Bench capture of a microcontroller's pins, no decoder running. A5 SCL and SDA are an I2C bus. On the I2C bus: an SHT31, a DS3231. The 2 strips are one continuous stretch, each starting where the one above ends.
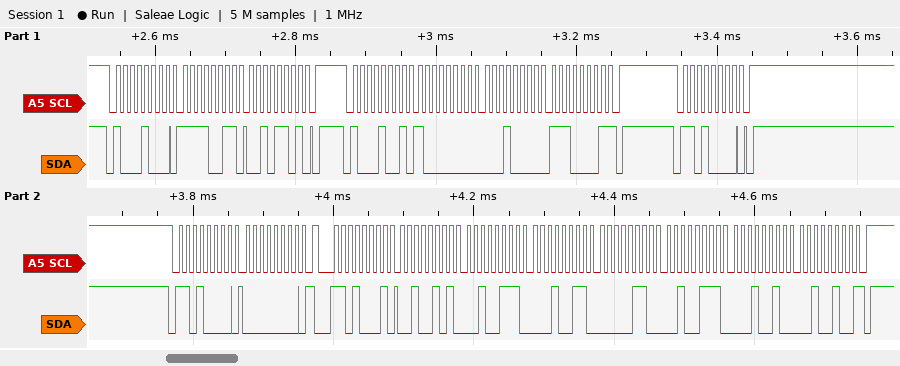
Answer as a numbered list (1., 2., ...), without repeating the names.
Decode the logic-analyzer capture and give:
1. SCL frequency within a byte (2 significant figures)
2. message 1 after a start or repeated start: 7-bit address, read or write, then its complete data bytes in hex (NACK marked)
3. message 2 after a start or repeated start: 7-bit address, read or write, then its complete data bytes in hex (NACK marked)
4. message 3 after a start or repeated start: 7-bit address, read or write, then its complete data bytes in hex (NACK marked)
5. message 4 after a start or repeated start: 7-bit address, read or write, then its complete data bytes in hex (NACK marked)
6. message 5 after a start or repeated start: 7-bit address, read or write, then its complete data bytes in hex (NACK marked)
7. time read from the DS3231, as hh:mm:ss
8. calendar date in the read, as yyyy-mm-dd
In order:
1. 100 kHz
2. 0x44 write: F3 2D
3. 0x44 read: 80 10 E1 NACK
4. 0x68 write
5. 0x68 write: 00
6. 0x68 read: 25 27 13 06 27 12 24 NACK
7. 13:27:25
8. 2024-12-27
